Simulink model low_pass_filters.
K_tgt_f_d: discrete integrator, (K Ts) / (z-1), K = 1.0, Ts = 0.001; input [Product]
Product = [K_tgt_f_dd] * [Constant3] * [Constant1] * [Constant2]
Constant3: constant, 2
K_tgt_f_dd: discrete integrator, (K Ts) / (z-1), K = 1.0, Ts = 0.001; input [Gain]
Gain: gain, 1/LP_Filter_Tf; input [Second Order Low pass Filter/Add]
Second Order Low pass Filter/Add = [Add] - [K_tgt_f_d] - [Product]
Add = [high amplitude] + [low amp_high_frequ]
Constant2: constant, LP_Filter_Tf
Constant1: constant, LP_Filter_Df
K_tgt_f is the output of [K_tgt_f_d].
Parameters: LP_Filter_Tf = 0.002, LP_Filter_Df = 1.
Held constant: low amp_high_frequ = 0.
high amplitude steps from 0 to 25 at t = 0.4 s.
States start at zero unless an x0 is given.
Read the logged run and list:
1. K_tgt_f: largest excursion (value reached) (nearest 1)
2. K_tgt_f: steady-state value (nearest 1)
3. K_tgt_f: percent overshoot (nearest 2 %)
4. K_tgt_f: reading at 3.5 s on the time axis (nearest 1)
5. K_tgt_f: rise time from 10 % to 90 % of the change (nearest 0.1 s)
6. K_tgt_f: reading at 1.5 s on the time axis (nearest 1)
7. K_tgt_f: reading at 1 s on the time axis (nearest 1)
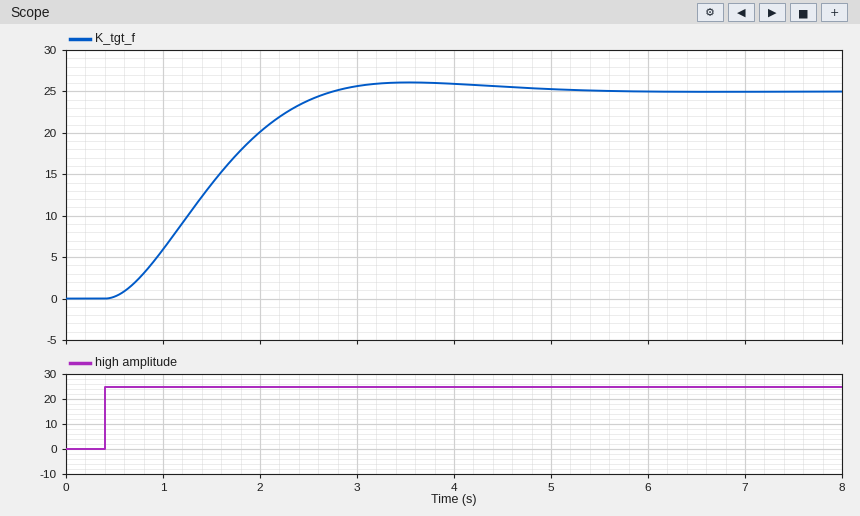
26
25
4 %
26
1.5 s
14
6
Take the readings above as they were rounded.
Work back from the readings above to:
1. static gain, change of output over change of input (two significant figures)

1.0
